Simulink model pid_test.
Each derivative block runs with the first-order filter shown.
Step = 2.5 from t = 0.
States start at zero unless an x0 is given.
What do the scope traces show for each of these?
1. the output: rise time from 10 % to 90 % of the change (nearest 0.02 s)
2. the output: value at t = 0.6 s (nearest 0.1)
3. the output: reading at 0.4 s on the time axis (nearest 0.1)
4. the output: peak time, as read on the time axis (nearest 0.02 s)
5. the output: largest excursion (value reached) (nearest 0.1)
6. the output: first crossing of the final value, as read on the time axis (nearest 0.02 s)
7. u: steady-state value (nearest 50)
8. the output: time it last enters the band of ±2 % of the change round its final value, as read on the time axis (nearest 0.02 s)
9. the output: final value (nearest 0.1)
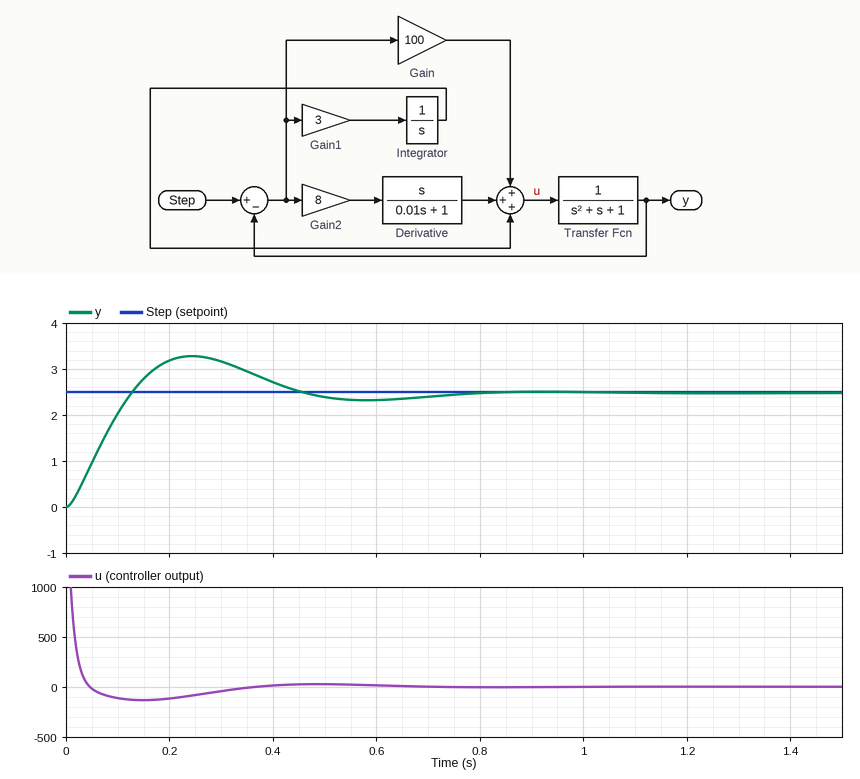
0.10 s
2.3
2.7
0.24 s
3.3
0.12 s
0
0.74 s
2.5
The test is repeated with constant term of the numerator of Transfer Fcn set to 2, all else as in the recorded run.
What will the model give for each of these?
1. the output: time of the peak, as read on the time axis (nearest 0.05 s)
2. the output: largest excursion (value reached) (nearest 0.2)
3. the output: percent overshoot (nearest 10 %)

0.15 s
3.2
30 %
